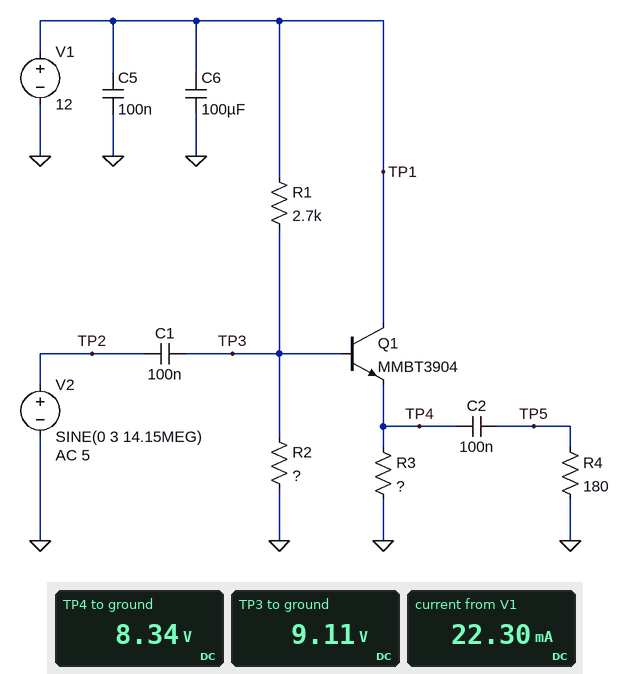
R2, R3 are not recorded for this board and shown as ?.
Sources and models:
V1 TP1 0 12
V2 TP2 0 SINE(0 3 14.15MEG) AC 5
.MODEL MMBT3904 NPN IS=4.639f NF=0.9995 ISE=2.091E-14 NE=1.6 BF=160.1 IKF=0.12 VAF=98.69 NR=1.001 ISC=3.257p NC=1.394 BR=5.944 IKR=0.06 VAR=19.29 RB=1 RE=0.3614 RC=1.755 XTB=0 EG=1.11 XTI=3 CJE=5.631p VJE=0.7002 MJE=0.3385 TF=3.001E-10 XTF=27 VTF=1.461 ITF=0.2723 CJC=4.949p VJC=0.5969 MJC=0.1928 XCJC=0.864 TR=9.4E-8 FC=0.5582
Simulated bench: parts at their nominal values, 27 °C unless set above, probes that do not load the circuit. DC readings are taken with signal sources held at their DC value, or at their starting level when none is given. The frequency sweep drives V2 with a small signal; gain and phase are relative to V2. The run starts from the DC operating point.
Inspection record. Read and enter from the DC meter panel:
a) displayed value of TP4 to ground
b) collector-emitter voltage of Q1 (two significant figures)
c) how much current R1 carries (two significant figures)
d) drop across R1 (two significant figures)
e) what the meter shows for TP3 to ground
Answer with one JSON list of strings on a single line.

["8.34 V", "3.7 V", "1.1 mA", "2.9 V", "9.11 V"]
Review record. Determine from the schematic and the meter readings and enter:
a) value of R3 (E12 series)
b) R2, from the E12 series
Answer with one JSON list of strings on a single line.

["390 Ω", "10 kΩ"]
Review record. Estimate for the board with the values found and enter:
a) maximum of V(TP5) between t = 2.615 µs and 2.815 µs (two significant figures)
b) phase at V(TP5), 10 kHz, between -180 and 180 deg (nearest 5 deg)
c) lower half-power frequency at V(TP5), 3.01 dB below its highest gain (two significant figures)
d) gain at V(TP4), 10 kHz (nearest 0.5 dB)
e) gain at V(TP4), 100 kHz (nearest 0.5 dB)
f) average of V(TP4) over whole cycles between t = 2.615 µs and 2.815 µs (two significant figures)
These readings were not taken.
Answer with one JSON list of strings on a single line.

["3.0 V", "45 deg", "8.9 kHz", "0 dB", "0 dB", "8.4 V"]
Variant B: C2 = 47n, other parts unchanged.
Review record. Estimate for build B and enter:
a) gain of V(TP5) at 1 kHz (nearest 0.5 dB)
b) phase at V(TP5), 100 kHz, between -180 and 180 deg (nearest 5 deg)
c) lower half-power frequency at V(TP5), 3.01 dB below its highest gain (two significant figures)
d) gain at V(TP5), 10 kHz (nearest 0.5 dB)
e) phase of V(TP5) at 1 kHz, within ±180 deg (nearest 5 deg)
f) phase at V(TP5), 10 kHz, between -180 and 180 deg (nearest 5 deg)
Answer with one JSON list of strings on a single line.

["-27.5 dB", "10 deg", "19 kHz", "-6.5 dB", "125 deg", "65 deg"]
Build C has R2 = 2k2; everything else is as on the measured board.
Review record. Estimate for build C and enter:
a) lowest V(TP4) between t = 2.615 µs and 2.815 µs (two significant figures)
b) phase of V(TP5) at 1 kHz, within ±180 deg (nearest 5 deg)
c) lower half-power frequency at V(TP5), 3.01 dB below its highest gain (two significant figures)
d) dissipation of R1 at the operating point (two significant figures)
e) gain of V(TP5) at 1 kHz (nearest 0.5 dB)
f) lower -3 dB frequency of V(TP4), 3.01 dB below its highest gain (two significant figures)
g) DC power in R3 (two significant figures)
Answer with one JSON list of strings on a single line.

["3.0 V", "135 deg", "9.0 kHz", "17 mW", "-23.5 dB", "1.3 kHz", "53 mW"]
